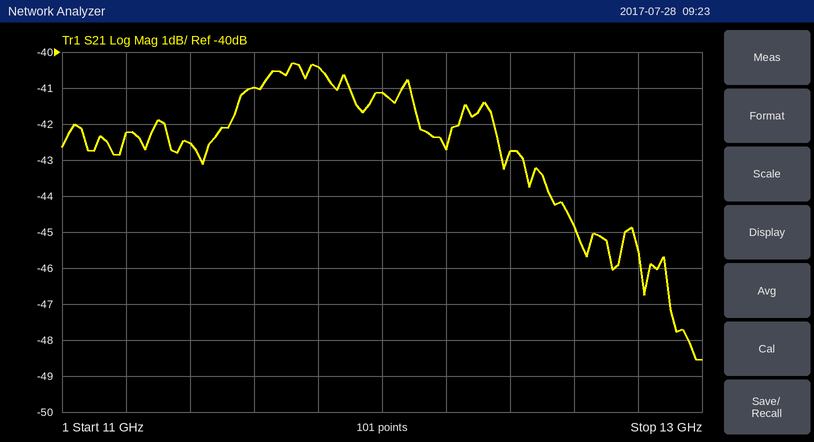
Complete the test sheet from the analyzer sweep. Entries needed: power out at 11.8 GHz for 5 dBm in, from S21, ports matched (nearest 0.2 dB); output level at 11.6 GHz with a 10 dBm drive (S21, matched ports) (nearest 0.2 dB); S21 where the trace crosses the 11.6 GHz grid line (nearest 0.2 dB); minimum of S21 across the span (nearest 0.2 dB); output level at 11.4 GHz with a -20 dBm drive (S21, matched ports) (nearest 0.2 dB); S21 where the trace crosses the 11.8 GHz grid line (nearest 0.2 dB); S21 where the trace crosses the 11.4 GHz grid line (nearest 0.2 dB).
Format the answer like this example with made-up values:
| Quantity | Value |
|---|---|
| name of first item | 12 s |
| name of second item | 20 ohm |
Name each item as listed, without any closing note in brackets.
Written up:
| Quantity | Value |
|---|---|
| power out at 11.8 GHz for 5 dBm in, from S21, ports matched | -35.4 dBm |
| output level at 11.6 GHz with a 10 dBm drive (S21, matched ports) | -31.0 dBm |
| S21 where the trace crosses the 11.6 GHz grid line | -41.0 dB |
| minimum of S21 across the span | -48.6 dB |
| output level at 11.4 GHz with a -20 dBm drive (S21, matched ports) | -62.6 dBm |
| S21 where the trace crosses the 11.8 GHz grid line | -40.4 dB |
| S21 where the trace crosses the 11.4 GHz grid line | -42.6 dB |
